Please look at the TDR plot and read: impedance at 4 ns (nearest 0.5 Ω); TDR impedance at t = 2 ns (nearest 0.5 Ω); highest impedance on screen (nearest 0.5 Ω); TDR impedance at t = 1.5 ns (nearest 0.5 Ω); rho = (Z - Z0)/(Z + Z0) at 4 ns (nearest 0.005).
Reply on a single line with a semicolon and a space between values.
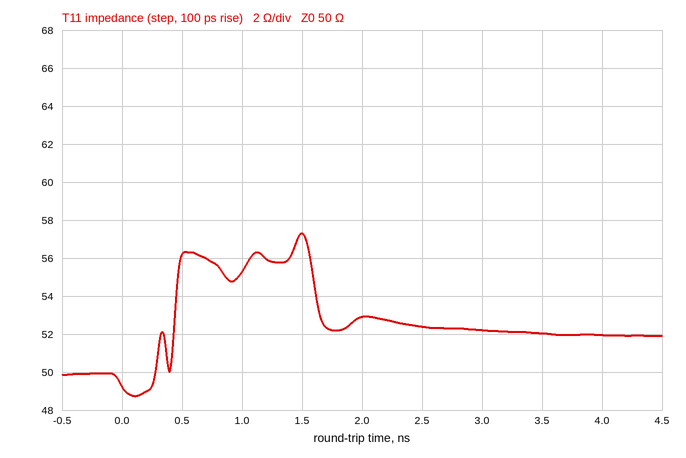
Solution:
52.0 Ω; 53.0 Ω; 57.5 Ω; 57.5 Ω; +0.020
